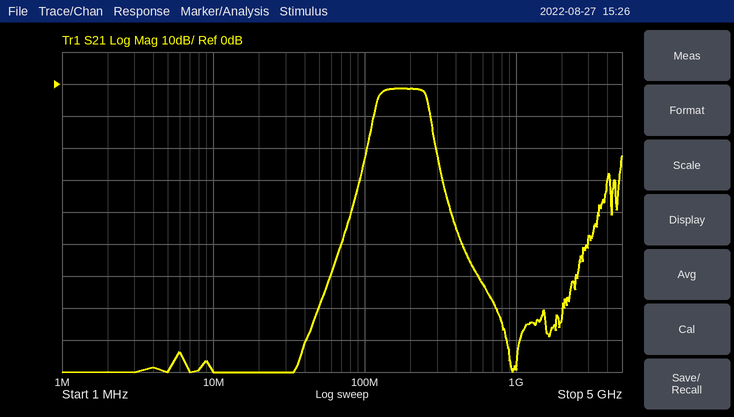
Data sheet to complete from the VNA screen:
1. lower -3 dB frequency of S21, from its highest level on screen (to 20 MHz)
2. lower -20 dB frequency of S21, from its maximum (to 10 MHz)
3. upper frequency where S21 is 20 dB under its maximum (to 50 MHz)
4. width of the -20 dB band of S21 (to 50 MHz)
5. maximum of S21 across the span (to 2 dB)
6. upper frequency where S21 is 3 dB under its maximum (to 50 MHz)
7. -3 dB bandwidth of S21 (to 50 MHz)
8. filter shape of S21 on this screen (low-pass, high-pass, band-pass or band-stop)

120 MHz
100 MHz
300 MHz
200 MHz
-2 dB
250 MHz
150 MHz
band-pass
